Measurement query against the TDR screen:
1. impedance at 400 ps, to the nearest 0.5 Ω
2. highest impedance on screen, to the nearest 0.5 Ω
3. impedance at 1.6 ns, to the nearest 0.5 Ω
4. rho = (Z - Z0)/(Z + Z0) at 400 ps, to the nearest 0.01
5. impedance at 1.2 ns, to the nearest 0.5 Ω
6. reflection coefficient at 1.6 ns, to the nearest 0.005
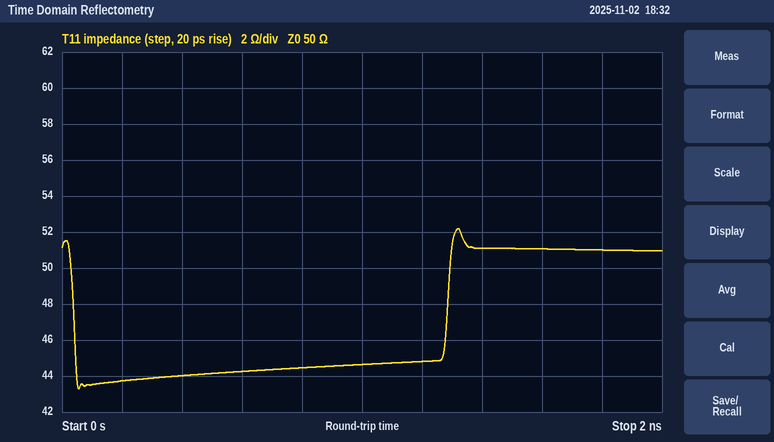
44.0 Ω
52.0 Ω
51.0 Ω
-0.06
45.0 Ω
+0.010
